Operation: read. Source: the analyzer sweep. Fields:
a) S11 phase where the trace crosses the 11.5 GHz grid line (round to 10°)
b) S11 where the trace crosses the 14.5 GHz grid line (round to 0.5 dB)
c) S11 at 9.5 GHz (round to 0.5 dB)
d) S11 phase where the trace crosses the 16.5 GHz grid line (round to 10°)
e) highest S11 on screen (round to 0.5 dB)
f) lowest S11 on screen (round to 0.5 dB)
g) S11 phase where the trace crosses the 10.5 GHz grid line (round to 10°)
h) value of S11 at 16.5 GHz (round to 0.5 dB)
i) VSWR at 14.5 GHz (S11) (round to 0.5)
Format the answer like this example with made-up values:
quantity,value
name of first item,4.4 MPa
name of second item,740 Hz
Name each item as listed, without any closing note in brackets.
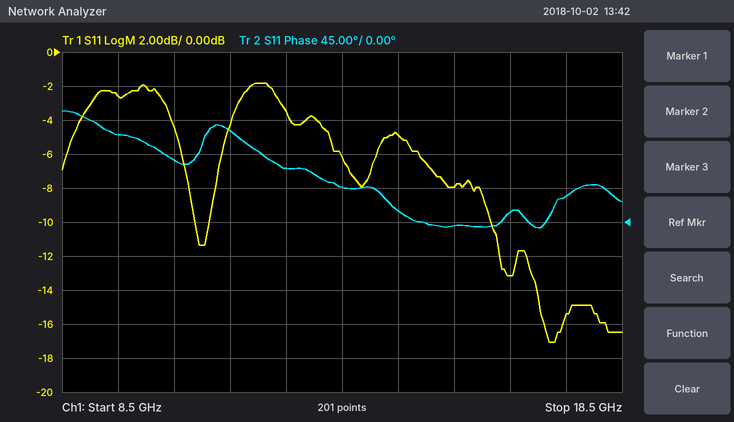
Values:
quantity,value
S11 phase where the trace crosses the 11.5 GHz grid line,120°
S11 where the trace crosses the 14.5 GHz grid line,-5.0 dB
S11 at 9.5 GHz,-2.5 dB
S11 phase where the trace crosses the 16.5 GHz grid line,10°
highest S11 on screen,-2.0 dB
lowest S11 on screen,-17.0 dB
S11 phase where the trace crosses the 10.5 GHz grid line,80°
value of S11 at 16.5 GHz,-13.0 dB
VSWR at 14.5 GHz (S11),3.5
